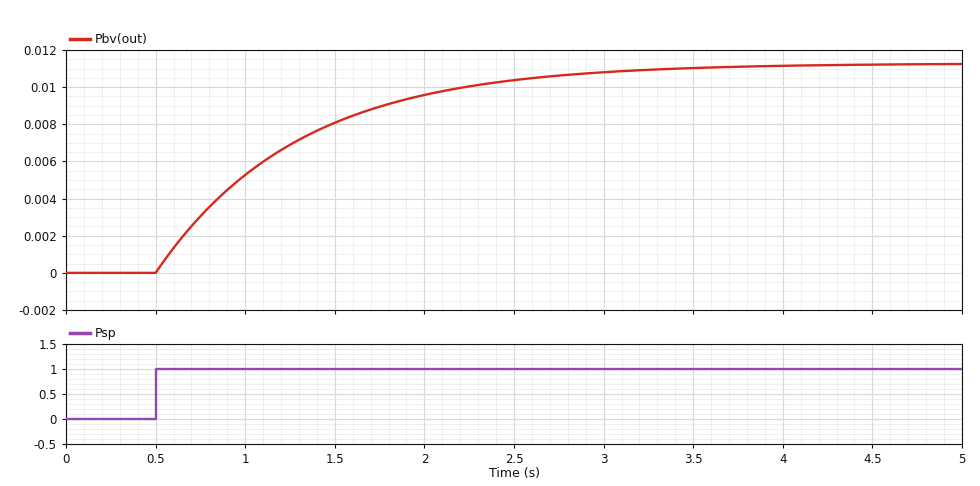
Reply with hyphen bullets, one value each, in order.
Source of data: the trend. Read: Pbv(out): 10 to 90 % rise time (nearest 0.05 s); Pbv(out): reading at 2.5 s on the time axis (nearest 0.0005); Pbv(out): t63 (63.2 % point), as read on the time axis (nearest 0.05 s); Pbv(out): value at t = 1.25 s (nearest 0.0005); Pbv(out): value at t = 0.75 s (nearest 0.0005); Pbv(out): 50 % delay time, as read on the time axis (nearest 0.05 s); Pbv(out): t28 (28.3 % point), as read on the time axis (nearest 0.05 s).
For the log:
- 1.75 s
- 0.0105
- 1.30 s
- 0.0070
- 0.0030
- 1.05 s
- 0.75 s
